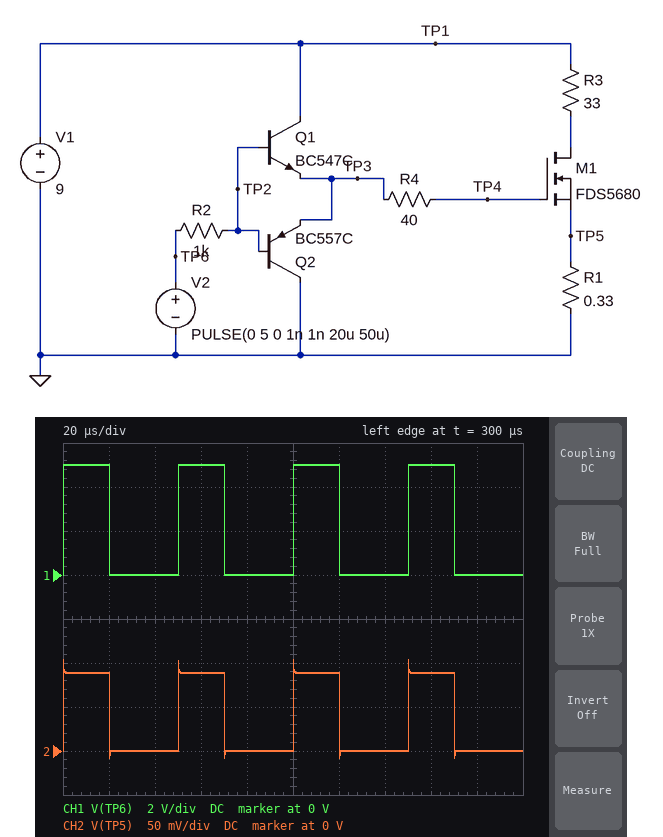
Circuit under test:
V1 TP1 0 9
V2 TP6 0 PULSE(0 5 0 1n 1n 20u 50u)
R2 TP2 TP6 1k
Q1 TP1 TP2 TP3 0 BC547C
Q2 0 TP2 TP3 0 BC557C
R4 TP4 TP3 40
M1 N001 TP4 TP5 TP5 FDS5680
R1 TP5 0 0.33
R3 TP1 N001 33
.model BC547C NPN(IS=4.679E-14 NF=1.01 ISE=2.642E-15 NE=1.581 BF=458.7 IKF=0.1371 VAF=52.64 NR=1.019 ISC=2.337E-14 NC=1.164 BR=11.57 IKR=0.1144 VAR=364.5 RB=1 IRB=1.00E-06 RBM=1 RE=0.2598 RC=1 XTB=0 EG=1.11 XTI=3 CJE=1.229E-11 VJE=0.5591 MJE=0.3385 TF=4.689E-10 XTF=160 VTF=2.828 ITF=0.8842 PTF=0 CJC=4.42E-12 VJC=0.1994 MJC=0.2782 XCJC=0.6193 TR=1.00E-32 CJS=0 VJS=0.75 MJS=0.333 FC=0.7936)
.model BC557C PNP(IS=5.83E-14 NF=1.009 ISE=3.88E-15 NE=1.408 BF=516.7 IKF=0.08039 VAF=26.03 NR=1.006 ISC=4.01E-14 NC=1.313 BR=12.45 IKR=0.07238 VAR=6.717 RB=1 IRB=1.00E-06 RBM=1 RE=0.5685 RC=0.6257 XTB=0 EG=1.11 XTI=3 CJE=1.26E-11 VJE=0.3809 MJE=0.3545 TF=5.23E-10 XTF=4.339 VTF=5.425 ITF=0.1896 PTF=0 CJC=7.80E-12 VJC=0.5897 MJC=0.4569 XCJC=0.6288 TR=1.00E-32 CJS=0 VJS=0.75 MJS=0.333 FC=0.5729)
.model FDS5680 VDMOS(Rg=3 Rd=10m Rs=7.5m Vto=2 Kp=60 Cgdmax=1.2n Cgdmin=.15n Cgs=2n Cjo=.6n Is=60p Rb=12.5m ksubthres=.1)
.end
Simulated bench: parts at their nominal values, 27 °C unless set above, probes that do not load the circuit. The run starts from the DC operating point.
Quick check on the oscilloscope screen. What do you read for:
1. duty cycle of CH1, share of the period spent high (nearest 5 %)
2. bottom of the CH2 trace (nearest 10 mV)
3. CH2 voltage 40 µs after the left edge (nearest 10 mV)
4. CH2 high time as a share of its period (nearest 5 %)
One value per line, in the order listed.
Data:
40 %
-10 mV
0 V
40 %
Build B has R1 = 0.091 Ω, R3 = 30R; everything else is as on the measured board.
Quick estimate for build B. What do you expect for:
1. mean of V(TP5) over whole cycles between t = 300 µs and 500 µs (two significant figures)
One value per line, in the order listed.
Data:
11 mV
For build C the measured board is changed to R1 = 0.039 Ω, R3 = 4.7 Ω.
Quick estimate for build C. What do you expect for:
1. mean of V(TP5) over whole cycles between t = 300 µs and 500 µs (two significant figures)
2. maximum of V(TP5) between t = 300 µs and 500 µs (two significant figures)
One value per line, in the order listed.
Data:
30 mV
75 mV
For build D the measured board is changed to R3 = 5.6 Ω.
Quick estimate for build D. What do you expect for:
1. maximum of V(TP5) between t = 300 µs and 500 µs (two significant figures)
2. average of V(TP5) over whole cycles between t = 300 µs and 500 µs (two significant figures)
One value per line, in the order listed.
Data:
510 mV
200 mV
